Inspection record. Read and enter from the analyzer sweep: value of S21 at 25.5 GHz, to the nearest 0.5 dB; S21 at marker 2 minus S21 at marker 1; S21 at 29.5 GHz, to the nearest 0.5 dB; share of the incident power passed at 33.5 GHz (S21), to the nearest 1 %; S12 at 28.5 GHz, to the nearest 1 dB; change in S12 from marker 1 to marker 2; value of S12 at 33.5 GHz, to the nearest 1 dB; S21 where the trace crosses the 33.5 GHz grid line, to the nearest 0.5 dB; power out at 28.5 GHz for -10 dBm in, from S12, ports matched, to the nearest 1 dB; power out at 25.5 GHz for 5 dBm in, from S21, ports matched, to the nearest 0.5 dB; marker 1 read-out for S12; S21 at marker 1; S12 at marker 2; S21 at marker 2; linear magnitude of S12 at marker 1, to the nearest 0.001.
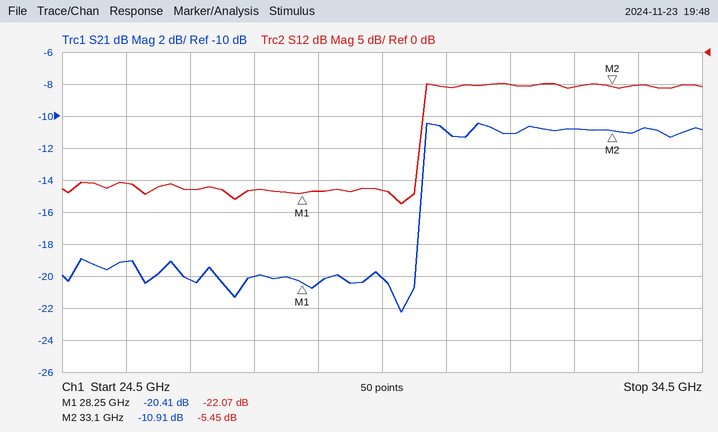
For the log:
-19.0 dB
9.50 dB
-20.0 dB
8 %
-22 dB
16.62 dB
-5 dB
-11.0 dB
-32 dBm
-14.0 dBm
-22.07 dB
-20.41 dB
-5.45 dB
-10.91 dB
0.079
